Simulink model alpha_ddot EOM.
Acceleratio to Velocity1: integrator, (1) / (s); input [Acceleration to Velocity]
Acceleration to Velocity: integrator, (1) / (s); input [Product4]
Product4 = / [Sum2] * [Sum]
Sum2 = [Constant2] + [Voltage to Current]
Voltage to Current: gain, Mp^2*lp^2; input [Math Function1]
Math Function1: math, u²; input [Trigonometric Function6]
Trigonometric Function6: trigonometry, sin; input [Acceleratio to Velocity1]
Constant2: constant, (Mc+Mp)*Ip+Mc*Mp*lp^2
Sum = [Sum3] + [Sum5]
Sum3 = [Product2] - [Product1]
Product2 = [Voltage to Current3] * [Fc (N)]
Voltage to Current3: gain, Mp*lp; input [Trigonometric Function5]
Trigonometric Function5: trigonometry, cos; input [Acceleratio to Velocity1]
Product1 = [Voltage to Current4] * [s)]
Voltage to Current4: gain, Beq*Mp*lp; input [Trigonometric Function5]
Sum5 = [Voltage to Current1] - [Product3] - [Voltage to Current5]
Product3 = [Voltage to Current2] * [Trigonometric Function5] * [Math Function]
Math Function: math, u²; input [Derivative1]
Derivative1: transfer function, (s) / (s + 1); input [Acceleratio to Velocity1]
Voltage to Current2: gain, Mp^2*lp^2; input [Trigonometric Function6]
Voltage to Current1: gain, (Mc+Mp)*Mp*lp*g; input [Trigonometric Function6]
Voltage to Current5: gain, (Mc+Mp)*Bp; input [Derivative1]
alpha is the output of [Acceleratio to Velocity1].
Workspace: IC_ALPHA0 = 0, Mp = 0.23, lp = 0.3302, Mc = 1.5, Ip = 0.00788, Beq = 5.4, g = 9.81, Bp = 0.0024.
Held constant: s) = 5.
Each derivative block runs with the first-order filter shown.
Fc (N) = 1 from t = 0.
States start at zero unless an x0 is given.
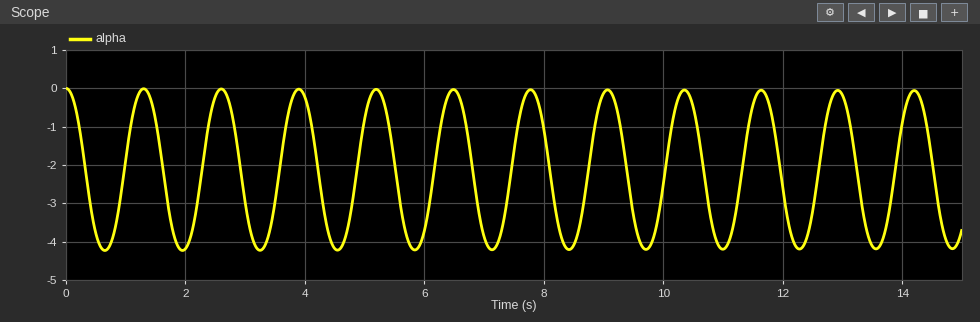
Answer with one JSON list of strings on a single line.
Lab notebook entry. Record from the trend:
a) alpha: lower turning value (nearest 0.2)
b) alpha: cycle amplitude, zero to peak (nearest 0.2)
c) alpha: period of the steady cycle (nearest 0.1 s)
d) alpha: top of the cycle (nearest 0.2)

["-4.2", "2.0", "1.3 s", "0.0"]
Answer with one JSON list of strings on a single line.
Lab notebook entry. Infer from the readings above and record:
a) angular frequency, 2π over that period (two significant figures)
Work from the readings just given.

["4.8 rad/s"]
